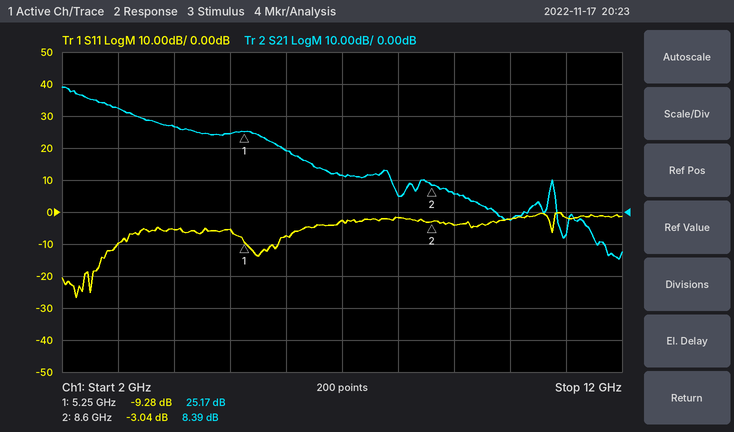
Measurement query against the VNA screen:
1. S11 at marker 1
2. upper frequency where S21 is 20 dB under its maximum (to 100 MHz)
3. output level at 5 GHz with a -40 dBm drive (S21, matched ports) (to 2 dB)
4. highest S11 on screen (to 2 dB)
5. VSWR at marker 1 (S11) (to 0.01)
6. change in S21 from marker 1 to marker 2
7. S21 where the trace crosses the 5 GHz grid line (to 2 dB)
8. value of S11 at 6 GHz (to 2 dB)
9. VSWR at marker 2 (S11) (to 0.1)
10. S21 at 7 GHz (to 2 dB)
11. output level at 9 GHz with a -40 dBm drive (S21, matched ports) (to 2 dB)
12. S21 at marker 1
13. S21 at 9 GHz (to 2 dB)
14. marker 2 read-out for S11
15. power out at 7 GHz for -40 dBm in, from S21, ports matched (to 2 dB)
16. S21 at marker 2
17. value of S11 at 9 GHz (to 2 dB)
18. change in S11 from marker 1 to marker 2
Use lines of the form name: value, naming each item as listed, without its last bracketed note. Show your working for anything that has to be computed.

S11 at marker 1: -9.28 dB
upper frequency where S21 is 20 dB under its maximum: 6.0 GHz
output level at 5 GHz with a -40 dBm drive (S21, matched ports): -40 dBm + (24 dB) = -16 dBm
highest S11 on screen: 0 dB
VSWR at marker 1 (S11): (1 + 0.3436)/(1 − 0.3436) ≈ 2.05
change in S21 from marker 1 to marker 2: 8.39 − (25.17) = -16.78 dB
S21 where the trace crosses the 5 GHz grid line: 24 dB
value of S11 at 6 GHz: -8 dB
VSWR at marker 2 (S11): (1 + 0.7047)/(1 − 0.7047) ≈ 5.8
S21 at 7 GHz: 12 dB
output level at 9 GHz with a -40 dBm drive (S21, matched ports): -40 dBm + (6 dB) = -34 dBm
S21 at marker 1: 25.17 dB
S21 at 9 GHz: 6 dB
marker 2 read-out for S11: -3.04 dB
power out at 7 GHz for -40 dBm in, from S21, ports matched: -40 dBm + (12 dB) = -28 dBm
S21 at marker 2: 8.39 dB
value of S11 at 9 GHz: -4 dB
change in S11 from marker 1 to marker 2: -3.04 − (-9.28) = 6.24 dB
